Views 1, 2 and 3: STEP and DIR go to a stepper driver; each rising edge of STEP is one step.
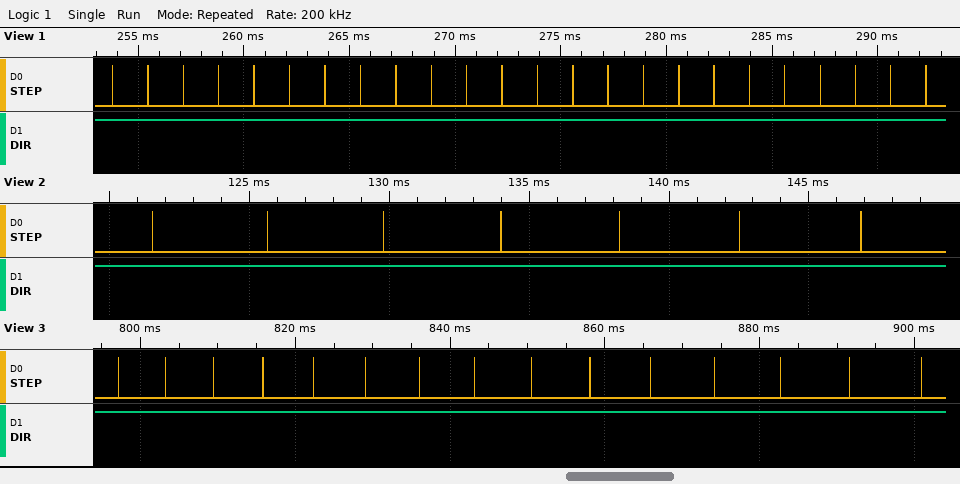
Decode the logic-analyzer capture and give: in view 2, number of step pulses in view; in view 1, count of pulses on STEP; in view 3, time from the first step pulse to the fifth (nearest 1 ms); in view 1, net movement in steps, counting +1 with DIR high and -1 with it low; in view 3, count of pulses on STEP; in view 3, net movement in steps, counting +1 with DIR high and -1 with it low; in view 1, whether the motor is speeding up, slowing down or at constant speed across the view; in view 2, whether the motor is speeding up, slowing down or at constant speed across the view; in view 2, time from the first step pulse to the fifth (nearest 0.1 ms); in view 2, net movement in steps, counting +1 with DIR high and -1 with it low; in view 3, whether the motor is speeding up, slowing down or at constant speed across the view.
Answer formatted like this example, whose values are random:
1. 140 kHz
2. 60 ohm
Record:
1. 7
2. 24
3. 25 ms
4. +24
5. 15
6. +15
7. constant speed
8. slowing down
9. 16.7 ms
10. +7
11. slowing down
